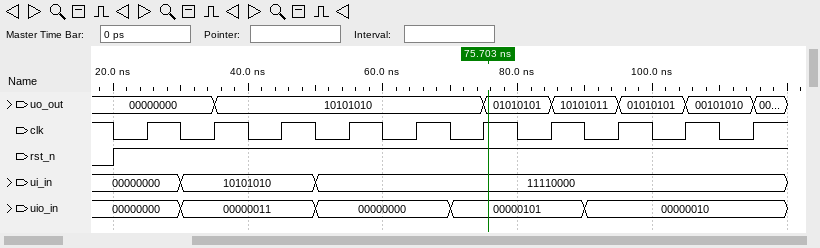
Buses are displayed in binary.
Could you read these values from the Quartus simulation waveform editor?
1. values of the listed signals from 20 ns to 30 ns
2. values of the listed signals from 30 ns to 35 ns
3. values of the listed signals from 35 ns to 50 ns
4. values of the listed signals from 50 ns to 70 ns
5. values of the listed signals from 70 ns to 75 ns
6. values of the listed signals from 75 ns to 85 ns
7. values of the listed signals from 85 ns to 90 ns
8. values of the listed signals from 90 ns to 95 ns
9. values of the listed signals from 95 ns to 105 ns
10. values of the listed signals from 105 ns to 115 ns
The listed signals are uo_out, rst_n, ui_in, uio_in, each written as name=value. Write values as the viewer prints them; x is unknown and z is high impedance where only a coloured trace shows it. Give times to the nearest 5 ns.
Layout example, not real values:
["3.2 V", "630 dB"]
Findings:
["uo_out=00000000, rst_n=1, ui_in=00000000, uio_in=00000000", "uo_out=00000000, rst_n=1, ui_in=10101010, uio_in=00000011", "uo_out=10101010, rst_n=1, ui_in=10101010, uio_in=00000011", "uo_out=10101010, rst_n=1, ui_in=11110000, uio_in=00000000", "uo_out=10101010, rst_n=1, ui_in=11110000, uio_in=00000101", "uo_out=01010101, rst_n=1, ui_in=11110000, uio_in=00000101", "uo_out=10101011, rst_n=1, ui_in=11110000, uio_in=00000101", "uo_out=10101011, rst_n=1, ui_in=11110000, uio_in=00000010", "uo_out=01010101, rst_n=1, ui_in=11110000, uio_in=00000010", "uo_out=00101010, rst_n=1, ui_in=11110000, uio_in=00000010"]
